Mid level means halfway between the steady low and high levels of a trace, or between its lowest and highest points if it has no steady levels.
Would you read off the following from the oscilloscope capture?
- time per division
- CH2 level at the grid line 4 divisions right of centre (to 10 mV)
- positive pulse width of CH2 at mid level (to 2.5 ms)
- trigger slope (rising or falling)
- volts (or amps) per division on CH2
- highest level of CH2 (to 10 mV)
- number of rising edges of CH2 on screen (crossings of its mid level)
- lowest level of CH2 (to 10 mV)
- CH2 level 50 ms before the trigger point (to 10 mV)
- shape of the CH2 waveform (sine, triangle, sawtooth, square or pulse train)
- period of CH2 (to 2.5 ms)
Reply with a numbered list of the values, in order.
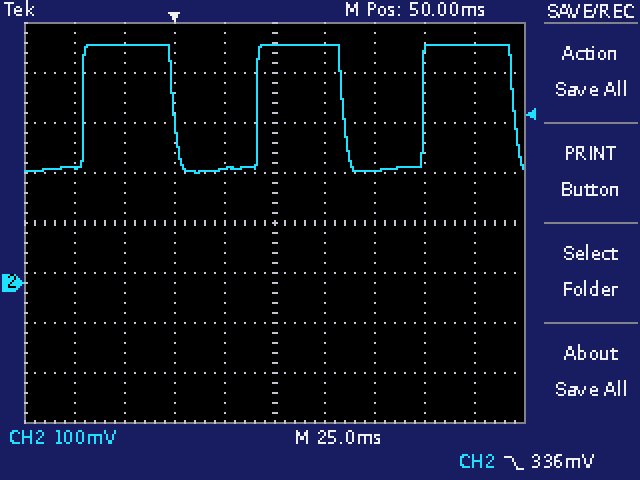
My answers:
1. 25 ms
2. 480 mV
3. 45.0 ms
4. falling
5. 100 mV
6. 480 mV
7. 3
8. 220 mV
9. 230 mV
10. square
11. 85.0 ms
